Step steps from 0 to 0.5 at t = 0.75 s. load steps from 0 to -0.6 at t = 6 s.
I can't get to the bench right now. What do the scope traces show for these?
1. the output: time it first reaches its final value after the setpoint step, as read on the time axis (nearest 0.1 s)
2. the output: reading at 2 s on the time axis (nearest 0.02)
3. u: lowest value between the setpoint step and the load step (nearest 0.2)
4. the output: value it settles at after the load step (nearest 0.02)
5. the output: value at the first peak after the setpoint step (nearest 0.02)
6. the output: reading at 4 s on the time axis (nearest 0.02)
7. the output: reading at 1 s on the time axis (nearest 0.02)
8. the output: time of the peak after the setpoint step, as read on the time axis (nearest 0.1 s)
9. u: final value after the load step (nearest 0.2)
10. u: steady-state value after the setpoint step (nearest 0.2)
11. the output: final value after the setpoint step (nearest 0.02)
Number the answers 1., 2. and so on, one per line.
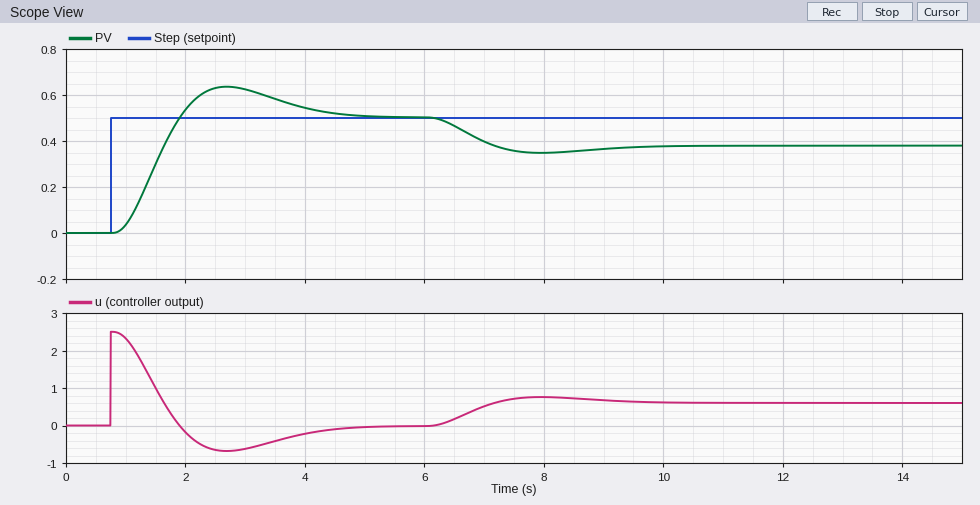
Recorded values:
1. 1.9 s
2. 0.54
3. -0.6
4. 0.38
5. 0.64
6. 0.54
7. 0.04
8. 2.7 s
9. 0.6
10. 0.0
11. 0.50
